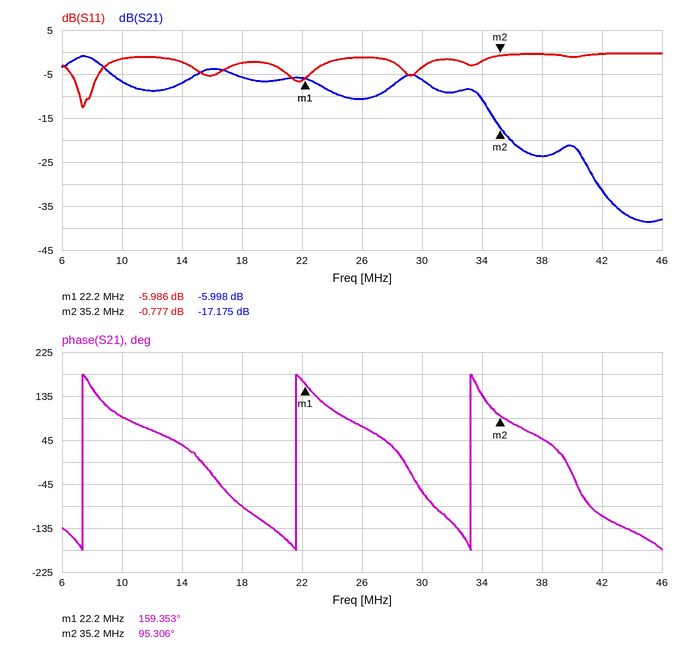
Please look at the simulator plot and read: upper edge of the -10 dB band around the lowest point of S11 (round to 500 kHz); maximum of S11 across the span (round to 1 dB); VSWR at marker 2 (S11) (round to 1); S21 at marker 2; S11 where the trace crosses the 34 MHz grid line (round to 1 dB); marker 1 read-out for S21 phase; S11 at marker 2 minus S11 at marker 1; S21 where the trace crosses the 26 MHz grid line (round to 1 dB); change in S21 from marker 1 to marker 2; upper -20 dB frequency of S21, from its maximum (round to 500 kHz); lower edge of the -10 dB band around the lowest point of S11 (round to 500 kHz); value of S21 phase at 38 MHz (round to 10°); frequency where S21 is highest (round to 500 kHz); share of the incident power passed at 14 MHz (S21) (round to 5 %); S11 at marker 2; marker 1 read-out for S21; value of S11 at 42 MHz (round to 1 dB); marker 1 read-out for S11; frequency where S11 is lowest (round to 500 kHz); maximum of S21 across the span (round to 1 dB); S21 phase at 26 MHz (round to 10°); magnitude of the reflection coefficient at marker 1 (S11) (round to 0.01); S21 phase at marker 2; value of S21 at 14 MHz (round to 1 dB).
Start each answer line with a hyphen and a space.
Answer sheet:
- 8.0 MHz
- 0 dB
- 22
- -17.175 dB
- -2 dB
- 159.353°
- 5.209 dB
- -11 dB
- -11.177 dB
- 36.0 MHz
- 7.0 MHz
- 50°
- 7.5 MHz
- 20 %
- -0.777 dB
- -5.998 dB
- 0 dB
- -5.986 dB
- 7.5 MHz
- -1 dB
- 70°
- 0.50
- 95.306°
- -7 dB
